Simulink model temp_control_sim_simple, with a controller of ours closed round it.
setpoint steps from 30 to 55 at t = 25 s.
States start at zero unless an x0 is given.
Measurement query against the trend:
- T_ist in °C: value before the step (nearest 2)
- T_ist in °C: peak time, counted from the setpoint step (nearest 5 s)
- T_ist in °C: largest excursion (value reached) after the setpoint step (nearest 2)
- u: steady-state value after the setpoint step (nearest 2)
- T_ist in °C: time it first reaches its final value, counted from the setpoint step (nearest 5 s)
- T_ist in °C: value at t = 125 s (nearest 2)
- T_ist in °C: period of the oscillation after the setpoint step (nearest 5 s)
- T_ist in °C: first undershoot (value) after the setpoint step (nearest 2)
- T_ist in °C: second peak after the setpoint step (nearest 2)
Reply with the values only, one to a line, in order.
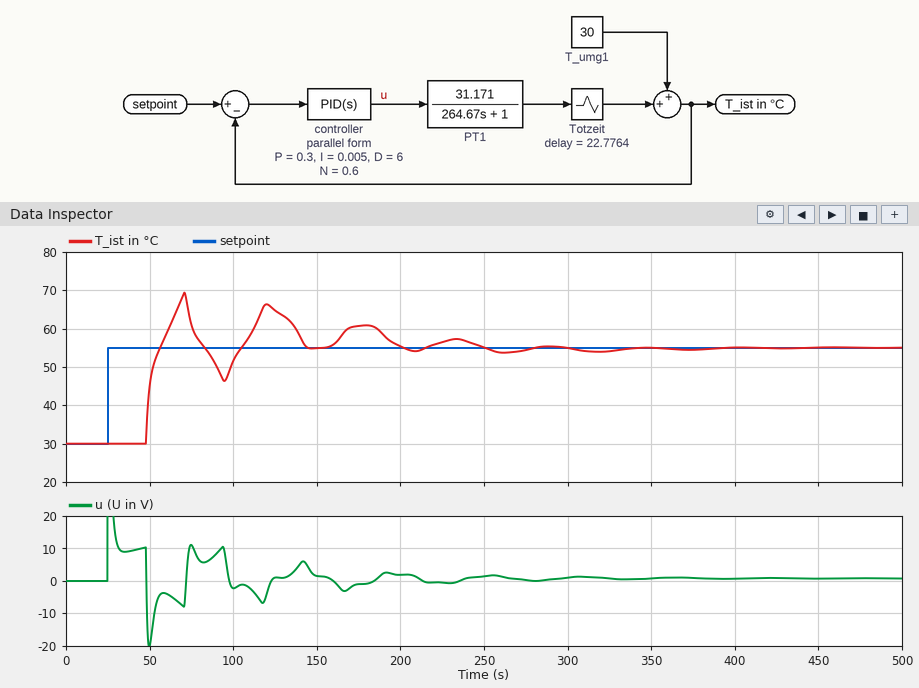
30
45 s
70
0
30 s
64
50 s
46
66
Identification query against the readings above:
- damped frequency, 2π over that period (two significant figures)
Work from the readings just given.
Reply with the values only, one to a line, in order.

0.13 rad/s
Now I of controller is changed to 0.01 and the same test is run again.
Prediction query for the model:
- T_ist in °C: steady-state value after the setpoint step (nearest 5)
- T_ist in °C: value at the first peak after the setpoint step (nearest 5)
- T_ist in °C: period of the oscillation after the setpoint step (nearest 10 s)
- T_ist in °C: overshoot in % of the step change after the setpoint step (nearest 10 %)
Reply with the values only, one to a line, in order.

55
75
50 s
70 %
